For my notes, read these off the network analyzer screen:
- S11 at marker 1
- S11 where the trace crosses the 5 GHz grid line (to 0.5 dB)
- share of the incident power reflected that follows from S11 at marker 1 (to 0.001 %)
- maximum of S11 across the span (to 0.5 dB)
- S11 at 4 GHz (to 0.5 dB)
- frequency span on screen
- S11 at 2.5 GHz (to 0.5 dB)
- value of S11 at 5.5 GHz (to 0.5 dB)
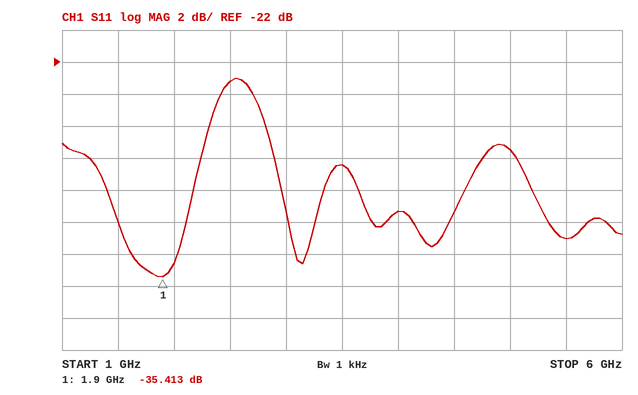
-35.413 dB
-27.5 dB
0.029 %
-23.0 dB
-31.5 dB
5 GHz
-23.0 dB
-33.0 dB
